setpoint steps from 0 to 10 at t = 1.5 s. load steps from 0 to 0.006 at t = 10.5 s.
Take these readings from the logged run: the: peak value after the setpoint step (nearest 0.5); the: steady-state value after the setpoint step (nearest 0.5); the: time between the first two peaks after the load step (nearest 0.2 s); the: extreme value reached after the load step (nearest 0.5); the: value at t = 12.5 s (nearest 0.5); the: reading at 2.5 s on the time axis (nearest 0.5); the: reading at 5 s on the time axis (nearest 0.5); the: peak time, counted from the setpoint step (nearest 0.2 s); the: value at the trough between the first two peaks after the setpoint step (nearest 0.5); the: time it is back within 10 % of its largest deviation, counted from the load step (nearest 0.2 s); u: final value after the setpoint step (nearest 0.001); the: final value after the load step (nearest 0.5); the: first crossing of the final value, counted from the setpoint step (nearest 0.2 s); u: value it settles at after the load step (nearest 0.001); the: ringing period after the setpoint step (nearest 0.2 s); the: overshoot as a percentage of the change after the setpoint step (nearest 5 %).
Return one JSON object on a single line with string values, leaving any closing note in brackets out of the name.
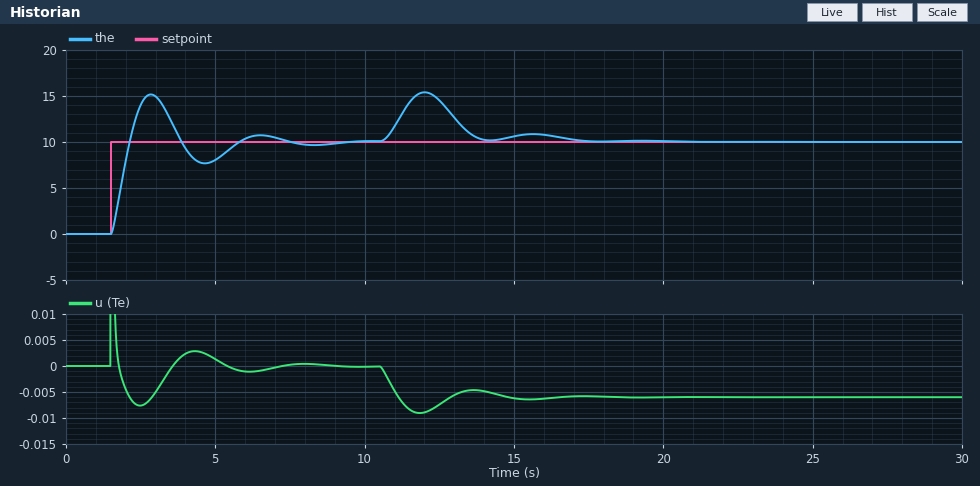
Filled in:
{"the: peak value after the setpoint step": "15.0", "the: steady-state value after the setpoint step": "10.0", "the: time between the first two peaks after the load step": "3.6 s", "the: extreme value reached after the load step": "15.5", "the: value at t = 12.5 s": "14.5", "the: reading at 2.5 s on the time axis": "14.0", "the: reading at 5 s on the time axis": "8.0", "the: peak time, counted from the setpoint step": "1.4 s", "the: value at the trough between the first two peaks after the setpoint step": "7.5", "the: time it is back within 10 % of its largest deviation, counted from the load step": "6.0 s", "u: final value after the setpoint step": "0.000", "the: final value after the load step": "10.0", "the: first crossing of the final value, counted from the setpoint step": "0.6 s", "u: value it settles at after the load step": "-0.006", "the: ringing period after the setpoint step": "3.6 s", "the: overshoot as a percentage of the change after the setpoint step": "50 %"}
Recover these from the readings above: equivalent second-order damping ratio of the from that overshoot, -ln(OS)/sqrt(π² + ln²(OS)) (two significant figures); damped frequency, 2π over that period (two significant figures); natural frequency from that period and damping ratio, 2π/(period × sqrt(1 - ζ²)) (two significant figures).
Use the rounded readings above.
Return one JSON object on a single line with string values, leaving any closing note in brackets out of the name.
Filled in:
{"equivalent second-order damping ratio of the from that overshoot, -ln(OS)/sqrt(π² + ln²(OS))": "0.22", "damped frequency, 2π over that period": "1.7 rad/s", "natural frequency from that period and damping ratio, 2π/(period × sqrt(1 - ζ²))": "1.8 rad/s"}
